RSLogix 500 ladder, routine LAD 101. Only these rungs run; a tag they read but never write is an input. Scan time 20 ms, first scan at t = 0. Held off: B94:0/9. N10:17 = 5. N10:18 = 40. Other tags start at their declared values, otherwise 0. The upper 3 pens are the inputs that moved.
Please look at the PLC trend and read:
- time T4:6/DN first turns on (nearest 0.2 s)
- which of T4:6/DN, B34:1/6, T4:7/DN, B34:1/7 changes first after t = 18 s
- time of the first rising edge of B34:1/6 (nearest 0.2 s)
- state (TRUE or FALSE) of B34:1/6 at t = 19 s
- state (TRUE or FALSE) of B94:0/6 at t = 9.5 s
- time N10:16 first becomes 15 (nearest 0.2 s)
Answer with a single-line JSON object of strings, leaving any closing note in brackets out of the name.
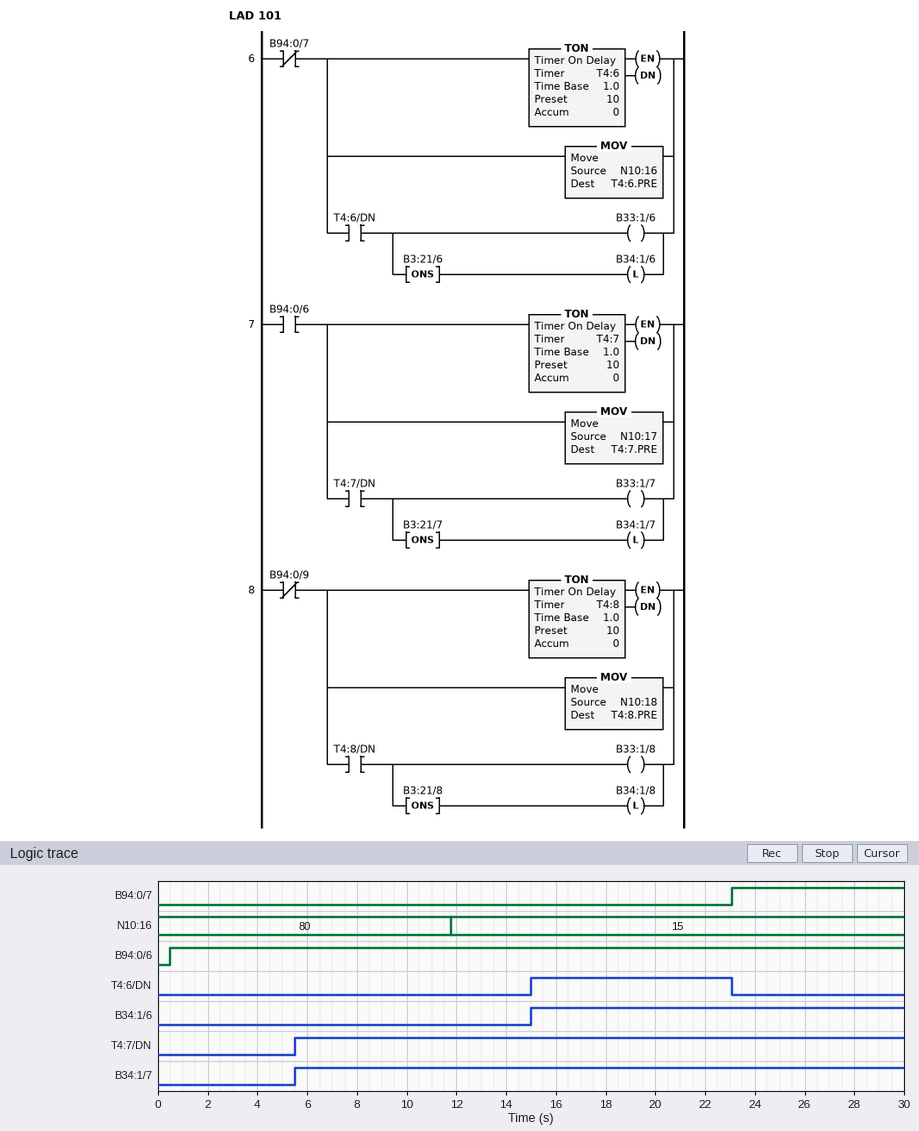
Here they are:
{"time T4:6/DN first turns on": "15.0 s", "which of T4:6/DN, B34:1/6, T4:7/DN, B34:1/7 changes first after t = 18 s": "T4:6/DN", "time of the first rising edge of B34:1/6": "15.0 s", "state (TRUE or FALSE) of B34:1/6 at t = 19 s": "TRUE", "state (TRUE or FALSE) of B94:0/6 at t = 9.5 s": "TRUE", "time N10:16 first becomes 15": "11.8 s"}
